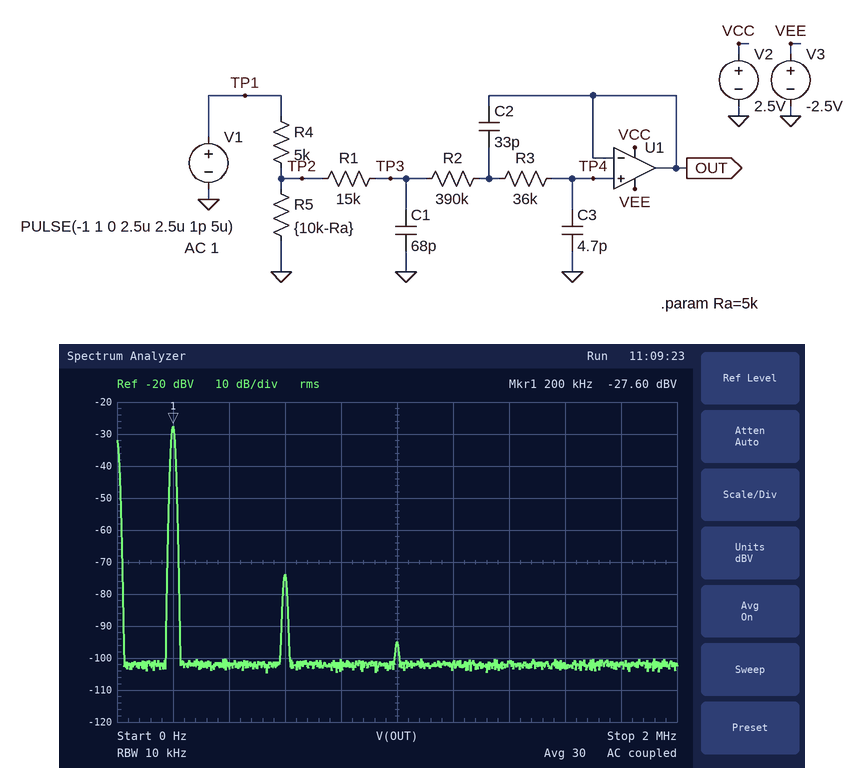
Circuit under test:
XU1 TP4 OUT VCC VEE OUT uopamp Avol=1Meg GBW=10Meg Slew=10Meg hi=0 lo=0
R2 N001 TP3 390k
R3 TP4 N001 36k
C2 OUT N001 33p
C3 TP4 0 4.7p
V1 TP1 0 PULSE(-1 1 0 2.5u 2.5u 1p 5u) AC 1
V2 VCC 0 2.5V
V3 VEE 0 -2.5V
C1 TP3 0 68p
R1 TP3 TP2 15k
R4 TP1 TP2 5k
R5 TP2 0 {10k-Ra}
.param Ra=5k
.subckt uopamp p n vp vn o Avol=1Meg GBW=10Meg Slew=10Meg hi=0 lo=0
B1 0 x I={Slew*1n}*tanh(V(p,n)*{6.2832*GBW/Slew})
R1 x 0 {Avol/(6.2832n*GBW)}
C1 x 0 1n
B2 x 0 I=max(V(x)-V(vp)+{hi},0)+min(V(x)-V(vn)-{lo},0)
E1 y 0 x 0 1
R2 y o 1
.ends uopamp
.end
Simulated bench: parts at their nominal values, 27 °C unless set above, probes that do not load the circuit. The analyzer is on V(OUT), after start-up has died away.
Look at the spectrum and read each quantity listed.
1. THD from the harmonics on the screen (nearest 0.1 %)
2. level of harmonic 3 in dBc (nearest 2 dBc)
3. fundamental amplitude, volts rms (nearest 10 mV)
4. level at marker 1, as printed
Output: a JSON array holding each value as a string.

["0.5 %", "-46 dBc", "40 mV", "-27.60 dBV"]
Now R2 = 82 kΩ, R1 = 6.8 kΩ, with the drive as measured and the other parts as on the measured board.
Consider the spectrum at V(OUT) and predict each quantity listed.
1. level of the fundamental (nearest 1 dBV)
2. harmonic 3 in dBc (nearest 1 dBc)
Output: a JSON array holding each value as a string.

["-11 dBV", "-44 dBc"]
